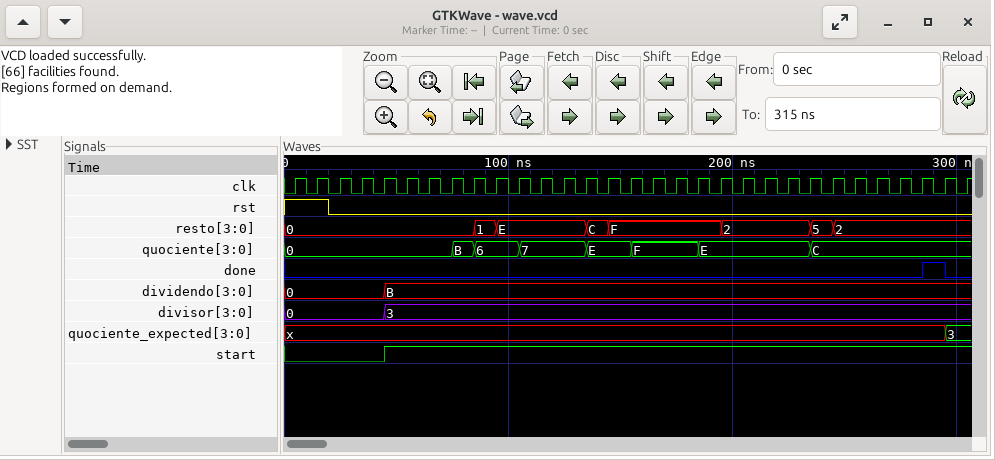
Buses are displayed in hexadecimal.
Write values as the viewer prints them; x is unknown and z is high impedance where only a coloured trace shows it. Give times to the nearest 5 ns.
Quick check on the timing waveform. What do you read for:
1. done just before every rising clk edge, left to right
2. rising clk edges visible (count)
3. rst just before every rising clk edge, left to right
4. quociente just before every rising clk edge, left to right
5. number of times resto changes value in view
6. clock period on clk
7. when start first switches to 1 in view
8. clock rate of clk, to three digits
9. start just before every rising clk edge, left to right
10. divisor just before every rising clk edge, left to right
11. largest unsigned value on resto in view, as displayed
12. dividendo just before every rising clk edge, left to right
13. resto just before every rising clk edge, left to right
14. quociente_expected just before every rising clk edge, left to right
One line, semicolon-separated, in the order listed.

0 0 0 0 0 0 0 0 0 0 0 0 0 0 0 0 0 0 0 0 0 0 0 0 0 0 0 0 0 1 0; 31; 1 1 0 0 0 0 0 0 0 0 0 0 0 0 0 0 0 0 0 0 0 0 0 0 0 0 0 0 0 0 0; 0, 0, 0, 0, 0, 0, 0, 0, B, 6, 6, 7, 7, 7, E, E, F, F, F, E, E, E, E, E, C, C, C, C, C, C, C; 7; 10 ns; 45 ns; 100 MHz; 0 0 0 0 0 1 1 1 1 1 1 1 1 1 1 1 1 1 1 1 1 1 1 1 1 1 1 1 1 1 1; 0, 0, 0, 0, 0, 3, 3, 3, 3, 3, 3, 3, 3, 3, 3, 3, 3, 3, 3, 3, 3, 3, 3, 3, 3, 3, 3, 3, 3, 3, 3; F; 0, 0, 0, 0, 0, B, B, B, B, B, B, B, B, B, B, B, B, B, B, B, B, B, B, B, B, B, B, B, B, B, B; 0, 0, 0, 0, 0, 0, 0, 0, 0, 1, E, E, E, E, C, F, F, F, F, F, 2, 2, 2, 2, 5, 2, 2, 2, 2, 2, 2; x, x, x, x, x, x, x, x, x, x, x, x, x, x, x, x, x, x, x, x, x, x, x, x, x, x, x, x, x, x, 3
